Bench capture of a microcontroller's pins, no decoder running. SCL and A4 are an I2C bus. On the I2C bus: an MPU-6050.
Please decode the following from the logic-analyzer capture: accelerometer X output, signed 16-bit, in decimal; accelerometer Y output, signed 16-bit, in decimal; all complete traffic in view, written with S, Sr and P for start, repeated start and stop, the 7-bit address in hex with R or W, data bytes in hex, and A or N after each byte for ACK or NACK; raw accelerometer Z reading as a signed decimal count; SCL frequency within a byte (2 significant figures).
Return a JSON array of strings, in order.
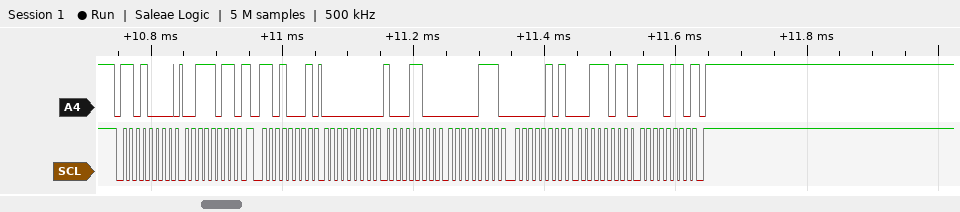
["140", "1797", "S 68W A 3B A Sr 68R A 00 A 8C A 07 A 05 A 3B A F6 N P", "15350", "100 kHz"]
